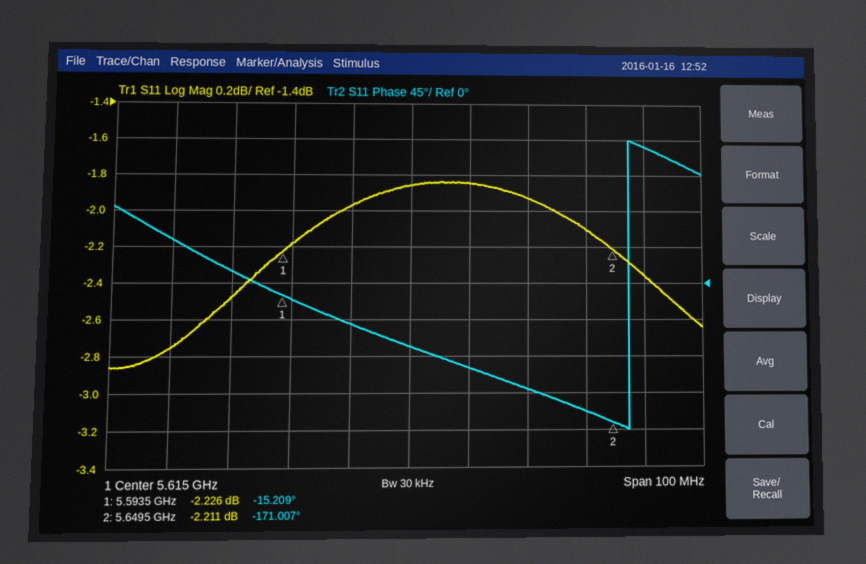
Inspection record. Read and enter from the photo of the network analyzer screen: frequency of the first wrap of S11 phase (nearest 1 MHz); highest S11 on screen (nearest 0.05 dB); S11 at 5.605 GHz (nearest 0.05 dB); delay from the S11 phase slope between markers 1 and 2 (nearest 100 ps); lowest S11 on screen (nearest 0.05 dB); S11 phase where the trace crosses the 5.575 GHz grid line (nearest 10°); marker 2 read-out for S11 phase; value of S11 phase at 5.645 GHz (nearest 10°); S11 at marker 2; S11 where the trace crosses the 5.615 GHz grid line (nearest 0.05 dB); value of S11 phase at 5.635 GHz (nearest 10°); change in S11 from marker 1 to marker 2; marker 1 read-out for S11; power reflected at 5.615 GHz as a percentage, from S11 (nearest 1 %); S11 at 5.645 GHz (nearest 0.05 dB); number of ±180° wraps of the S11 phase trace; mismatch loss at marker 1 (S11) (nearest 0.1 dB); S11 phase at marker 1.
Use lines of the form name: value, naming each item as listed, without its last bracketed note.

frequency of the first wrap of S11 phase: 5.652 GHz
highest S11 on screen: -1.85 dB
S11 at 5.605 GHz: -1.95 dB
delay from the S11 phase slope between markers 1 and 2: 7.7 ns
lowest S11 on screen: -2.85 dB
S11 phase where the trace crosses the 5.575 GHz grid line: 50°
marker 2 read-out for S11 phase: -171.007°
value of S11 phase at 5.645 GHz: -160°
S11 at marker 2: -2.211 dB
S11 where the trace crosses the 5.615 GHz grid line: -1.85 dB
value of S11 phase at 5.635 GHz: -130°
change in S11 from marker 1 to marker 2: 0.015 dB
marker 1 read-out for S11: -2.226 dB
power reflected at 5.615 GHz as a percentage, from S11: 65 %
S11 at 5.645 GHz: -2.10 dB
number of ±180° wraps of the S11 phase trace: 1
mismatch loss at marker 1 (S11): 4.0 dB
S11 phase at marker 1: -15.209°
